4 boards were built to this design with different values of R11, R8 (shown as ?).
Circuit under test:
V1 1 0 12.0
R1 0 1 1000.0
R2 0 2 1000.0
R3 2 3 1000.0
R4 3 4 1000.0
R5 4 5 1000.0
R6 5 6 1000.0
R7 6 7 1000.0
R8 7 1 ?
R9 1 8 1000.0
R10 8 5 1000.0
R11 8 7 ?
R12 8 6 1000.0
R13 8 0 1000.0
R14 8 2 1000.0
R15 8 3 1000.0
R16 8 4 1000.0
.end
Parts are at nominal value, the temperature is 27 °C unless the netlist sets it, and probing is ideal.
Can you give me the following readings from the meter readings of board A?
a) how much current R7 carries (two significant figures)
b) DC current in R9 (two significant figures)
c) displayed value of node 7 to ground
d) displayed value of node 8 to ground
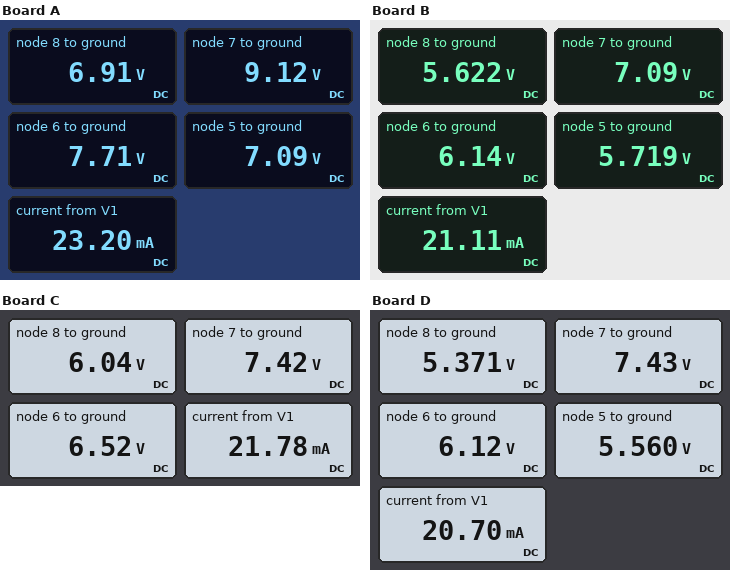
1.4 mA
5.1 mA
9.12 V
6.91 V
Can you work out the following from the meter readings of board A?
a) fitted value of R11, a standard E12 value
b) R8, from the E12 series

470 Ω
470 Ω
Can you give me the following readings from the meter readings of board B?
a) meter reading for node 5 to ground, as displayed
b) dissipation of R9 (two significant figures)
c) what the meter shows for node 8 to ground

5.719 V
41 mW
5.622 V
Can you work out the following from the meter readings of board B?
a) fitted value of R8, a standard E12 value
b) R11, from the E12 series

1.8 kΩ
820 Ω
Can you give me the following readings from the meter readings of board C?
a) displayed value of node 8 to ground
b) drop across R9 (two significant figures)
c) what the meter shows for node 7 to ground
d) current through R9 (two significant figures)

6.04 V
6.0 V
7.42 V
6.0 mA
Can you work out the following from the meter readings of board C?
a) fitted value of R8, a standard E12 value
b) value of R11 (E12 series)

1.2 kΩ
470 Ω
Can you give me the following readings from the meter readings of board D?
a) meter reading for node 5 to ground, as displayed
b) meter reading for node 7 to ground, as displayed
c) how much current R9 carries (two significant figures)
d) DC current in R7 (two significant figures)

5.560 V
7.43 V
6.6 mA
1.3 mA
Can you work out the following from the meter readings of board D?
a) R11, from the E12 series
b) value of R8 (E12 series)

2.7 kΩ
2.2 kΩ
